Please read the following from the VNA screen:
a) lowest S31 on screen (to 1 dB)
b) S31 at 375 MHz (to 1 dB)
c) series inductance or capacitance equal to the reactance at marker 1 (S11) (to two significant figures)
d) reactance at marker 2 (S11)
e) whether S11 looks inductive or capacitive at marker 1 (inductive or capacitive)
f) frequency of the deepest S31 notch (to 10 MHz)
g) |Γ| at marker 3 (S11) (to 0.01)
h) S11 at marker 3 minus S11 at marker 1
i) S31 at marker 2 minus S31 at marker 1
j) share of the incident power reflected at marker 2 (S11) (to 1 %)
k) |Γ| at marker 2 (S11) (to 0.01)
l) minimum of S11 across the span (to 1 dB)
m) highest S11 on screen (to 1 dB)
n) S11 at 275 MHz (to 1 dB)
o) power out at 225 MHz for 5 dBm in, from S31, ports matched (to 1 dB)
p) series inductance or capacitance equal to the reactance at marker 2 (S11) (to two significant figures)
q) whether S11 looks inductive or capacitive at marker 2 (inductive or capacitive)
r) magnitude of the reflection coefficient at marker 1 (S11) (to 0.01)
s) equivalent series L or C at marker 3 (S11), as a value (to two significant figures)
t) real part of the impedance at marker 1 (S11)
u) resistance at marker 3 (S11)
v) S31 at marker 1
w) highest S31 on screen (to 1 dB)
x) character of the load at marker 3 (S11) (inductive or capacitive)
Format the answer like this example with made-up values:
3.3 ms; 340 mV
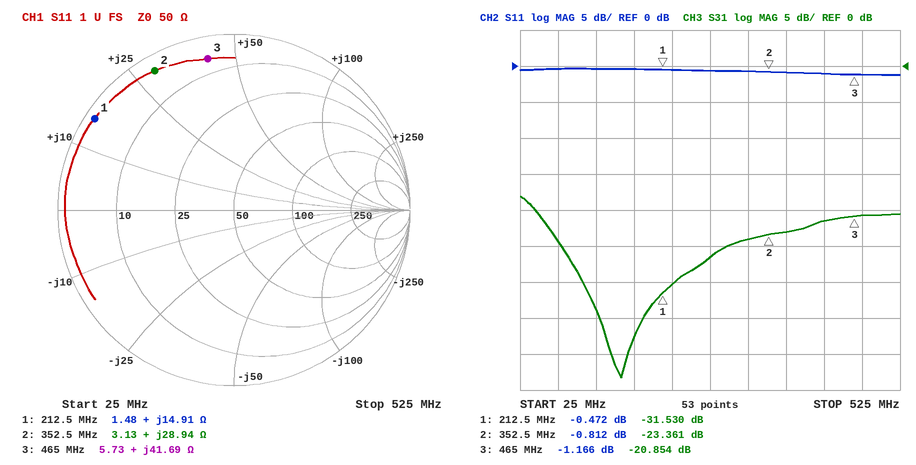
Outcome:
-43 dB; -23 dB; 11 nH; +28.94 Ω; inductive; 160 MHz; 0.87; -0.694 dB; 8.169 dB; 83 %; 0.91; -1 dB; 0 dB; -1 dB; -25 dBm; 13 nH; inductive; 0.95; 14 nH; 1.48 Ω; 5.73 Ω; -31.530 dB; -18 dB; inductive
